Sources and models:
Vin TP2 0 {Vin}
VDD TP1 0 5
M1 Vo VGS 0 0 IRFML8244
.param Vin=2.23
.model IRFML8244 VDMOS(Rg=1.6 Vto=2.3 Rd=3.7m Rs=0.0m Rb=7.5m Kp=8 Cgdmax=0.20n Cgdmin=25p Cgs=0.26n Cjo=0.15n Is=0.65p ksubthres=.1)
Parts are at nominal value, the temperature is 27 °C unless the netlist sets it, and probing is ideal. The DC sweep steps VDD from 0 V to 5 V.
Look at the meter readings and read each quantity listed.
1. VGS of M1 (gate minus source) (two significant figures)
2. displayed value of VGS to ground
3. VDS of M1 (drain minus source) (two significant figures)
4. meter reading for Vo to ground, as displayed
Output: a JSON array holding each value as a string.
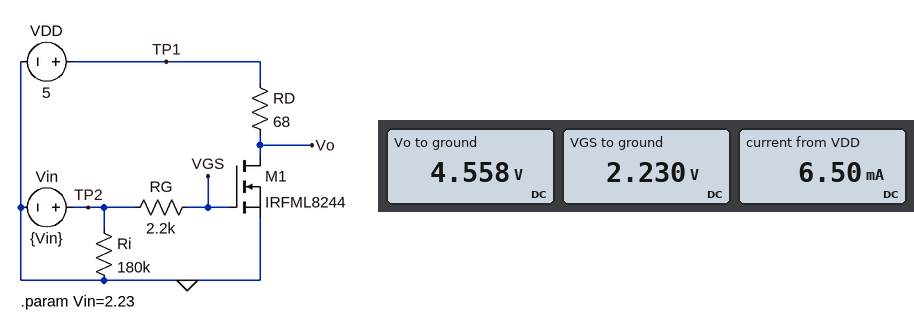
["2.2 V", "2.230 V", "4.6 V", "4.558 V"]
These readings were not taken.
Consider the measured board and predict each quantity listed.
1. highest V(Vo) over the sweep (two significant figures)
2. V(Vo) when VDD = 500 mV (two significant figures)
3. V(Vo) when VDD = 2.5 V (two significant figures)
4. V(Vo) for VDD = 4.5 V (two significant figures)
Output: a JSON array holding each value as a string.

["4.6 V", "58 mV", "2.1 V", "4.1 V"]
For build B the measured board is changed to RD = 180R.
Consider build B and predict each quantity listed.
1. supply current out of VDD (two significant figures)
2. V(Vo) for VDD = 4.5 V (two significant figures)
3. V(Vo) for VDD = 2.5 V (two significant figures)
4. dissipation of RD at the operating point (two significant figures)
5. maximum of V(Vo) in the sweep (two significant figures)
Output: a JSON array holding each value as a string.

["6.5 mA", "3.3 V", "1.3 V", "7.6 mW", "3.8 V"]
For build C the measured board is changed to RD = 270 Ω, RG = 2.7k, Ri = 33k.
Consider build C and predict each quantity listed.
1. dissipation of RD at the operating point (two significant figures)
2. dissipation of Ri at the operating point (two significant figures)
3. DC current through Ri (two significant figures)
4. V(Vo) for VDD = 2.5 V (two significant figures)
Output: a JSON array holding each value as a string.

["11 mW", "150 µW", "68 µA", "740 mV"]
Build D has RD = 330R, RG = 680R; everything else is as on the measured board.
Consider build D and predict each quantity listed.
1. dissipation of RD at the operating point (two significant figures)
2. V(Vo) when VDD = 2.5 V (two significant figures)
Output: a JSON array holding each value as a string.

["14 mW", "350 mV"]
